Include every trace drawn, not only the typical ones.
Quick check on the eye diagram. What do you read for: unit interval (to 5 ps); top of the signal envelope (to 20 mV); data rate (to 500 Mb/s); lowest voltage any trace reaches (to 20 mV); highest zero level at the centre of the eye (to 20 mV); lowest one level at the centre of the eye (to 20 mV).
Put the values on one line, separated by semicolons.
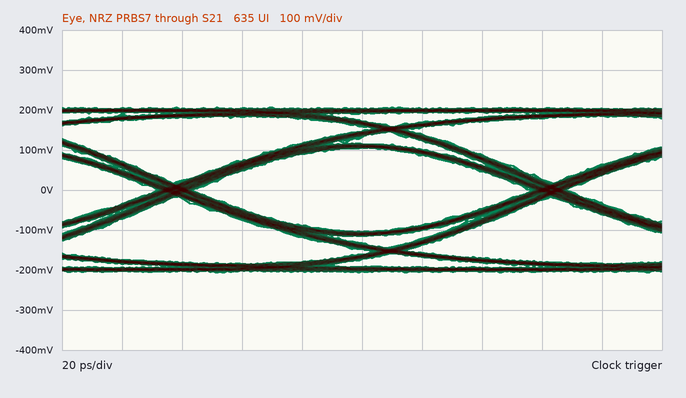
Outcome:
125 ps; 200 mV; 8.0 Gb/s; -200 mV; -100 mV; 100 mV
